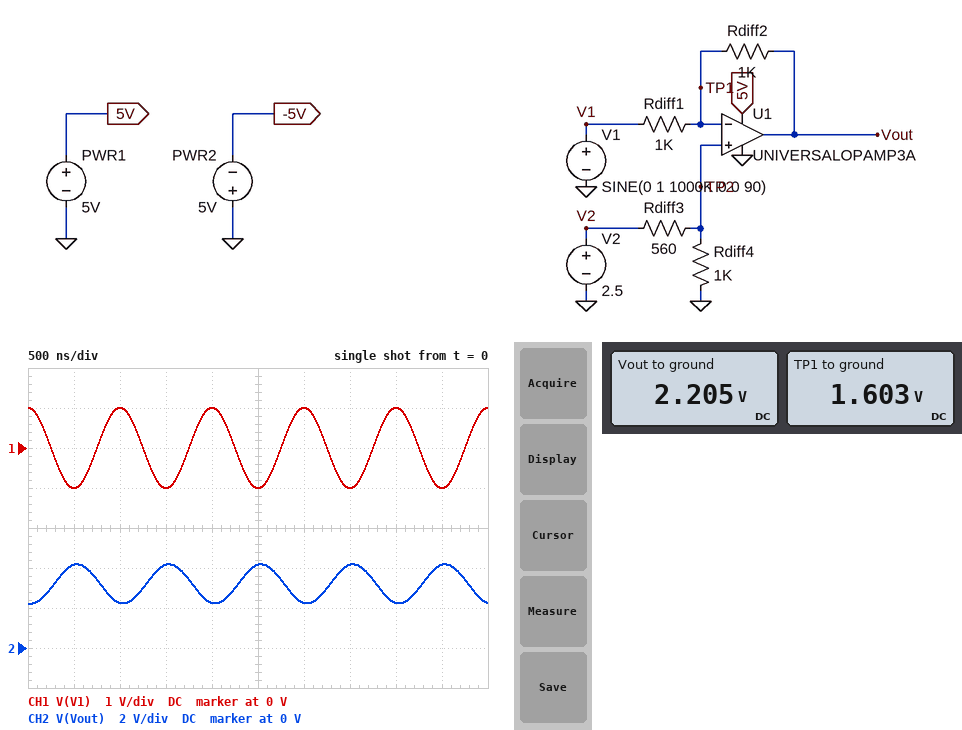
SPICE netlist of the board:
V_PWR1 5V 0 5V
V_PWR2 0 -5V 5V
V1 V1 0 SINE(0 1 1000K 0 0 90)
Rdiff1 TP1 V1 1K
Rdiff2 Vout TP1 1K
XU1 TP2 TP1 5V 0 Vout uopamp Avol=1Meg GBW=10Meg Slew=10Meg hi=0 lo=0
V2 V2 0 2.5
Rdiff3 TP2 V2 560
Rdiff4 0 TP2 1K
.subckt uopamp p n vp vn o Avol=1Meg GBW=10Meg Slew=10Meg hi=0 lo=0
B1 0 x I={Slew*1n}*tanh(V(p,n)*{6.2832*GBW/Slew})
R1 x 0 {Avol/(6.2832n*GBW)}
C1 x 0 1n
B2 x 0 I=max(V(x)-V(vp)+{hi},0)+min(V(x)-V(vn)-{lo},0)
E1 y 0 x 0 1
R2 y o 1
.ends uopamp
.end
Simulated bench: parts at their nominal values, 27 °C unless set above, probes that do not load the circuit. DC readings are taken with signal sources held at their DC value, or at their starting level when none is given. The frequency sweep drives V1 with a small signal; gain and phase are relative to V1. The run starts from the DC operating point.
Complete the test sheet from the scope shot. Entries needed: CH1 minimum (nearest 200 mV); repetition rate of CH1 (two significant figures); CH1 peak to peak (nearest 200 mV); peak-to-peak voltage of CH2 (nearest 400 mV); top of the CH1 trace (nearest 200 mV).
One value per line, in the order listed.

-1.0 V
1.0 MHz
2.0 V
2.0 V
1.0 V
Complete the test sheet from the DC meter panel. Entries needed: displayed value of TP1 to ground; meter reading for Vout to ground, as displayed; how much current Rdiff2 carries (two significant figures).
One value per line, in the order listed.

1.603 V
2.205 V
600 µA
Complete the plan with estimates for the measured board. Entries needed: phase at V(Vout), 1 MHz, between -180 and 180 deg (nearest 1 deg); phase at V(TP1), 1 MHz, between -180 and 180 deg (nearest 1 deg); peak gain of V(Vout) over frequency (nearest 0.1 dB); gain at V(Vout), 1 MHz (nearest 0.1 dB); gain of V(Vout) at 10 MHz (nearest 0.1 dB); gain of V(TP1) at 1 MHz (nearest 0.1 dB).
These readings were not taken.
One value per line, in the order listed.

169 deg
79 deg
0 dB
-0.2 dB
-7.0 dB
-20.2 dB
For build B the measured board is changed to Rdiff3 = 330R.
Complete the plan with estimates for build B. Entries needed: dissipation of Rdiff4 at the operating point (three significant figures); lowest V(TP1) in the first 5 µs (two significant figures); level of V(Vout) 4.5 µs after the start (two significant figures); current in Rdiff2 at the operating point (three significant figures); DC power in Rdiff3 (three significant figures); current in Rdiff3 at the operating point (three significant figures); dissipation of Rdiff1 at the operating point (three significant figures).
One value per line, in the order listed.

3.53 mW
1.8 V
4.7 V
880 µA
1.17 mW
1.88 mA
774 µW
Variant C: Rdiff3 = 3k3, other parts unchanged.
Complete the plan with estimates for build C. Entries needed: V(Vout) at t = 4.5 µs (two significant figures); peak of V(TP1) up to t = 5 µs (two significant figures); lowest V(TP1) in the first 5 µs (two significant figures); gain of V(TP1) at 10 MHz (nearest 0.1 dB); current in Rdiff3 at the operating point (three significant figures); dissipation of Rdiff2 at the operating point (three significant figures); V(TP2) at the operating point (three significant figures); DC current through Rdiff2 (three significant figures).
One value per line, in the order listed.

2.1 V
690 mV
470 mV
-7.0 dB
581 µA
175 µW
581 mV
419 µA
